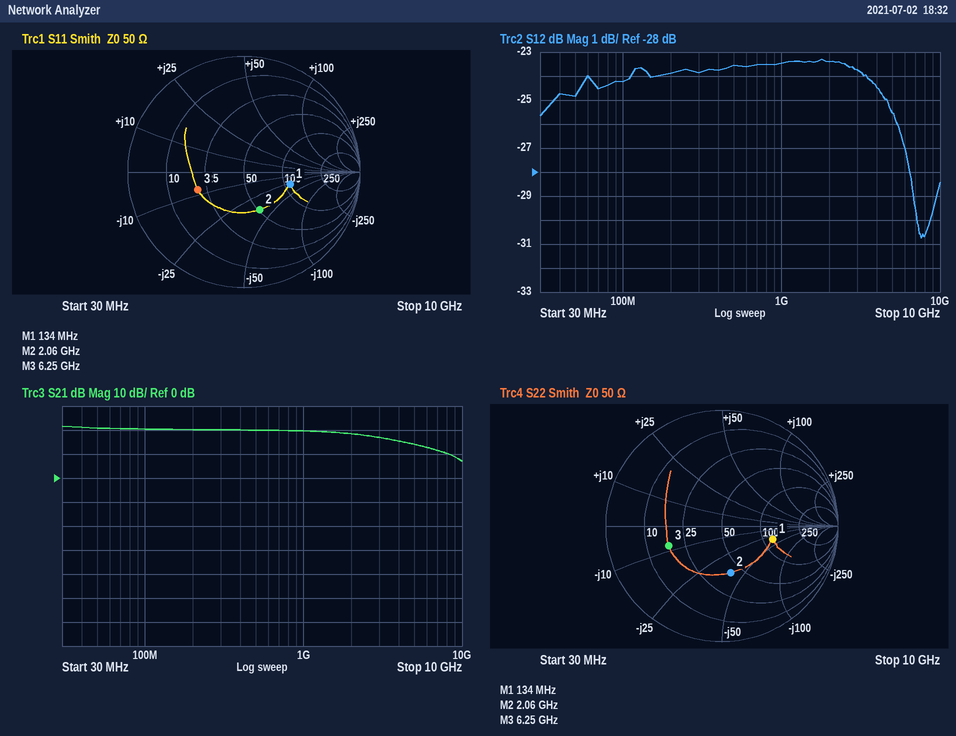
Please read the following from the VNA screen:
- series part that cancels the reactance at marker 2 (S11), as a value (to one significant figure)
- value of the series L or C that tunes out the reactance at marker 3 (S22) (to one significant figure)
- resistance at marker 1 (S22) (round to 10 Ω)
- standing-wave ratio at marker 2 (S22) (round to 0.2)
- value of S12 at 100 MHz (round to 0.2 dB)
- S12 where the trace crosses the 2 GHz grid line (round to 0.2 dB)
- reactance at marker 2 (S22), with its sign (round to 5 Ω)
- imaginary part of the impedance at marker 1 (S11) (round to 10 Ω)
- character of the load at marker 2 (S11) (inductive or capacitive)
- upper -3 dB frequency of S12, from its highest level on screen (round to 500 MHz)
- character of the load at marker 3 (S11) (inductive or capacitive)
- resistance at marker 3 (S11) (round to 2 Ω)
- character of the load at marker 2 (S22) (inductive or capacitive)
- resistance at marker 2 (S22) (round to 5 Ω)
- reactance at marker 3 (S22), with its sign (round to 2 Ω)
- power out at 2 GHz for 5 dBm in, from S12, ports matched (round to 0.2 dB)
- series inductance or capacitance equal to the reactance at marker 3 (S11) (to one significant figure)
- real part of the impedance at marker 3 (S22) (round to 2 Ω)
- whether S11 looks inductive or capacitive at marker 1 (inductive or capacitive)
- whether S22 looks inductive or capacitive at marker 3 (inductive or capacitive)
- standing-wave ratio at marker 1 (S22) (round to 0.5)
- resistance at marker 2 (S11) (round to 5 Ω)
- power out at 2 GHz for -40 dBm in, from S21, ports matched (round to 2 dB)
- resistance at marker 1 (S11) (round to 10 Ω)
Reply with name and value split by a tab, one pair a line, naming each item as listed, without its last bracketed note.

series part that cancels the reactance at marker 2 (S11), as a value	3 nH
value of the series L or C that tunes out the reactance at marker 3 (S22)	200 pH
resistance at marker 1 (S22)	120 Ω
standing-wave ratio at marker 2 (S22)	2.4
value of S12 at 100 MHz	-24.2 dB
S12 where the trace crosses the 2 GHz grid line	-23.4 dB
reactance at marker 2 (S22), with its sign	-40 Ω
imaginary part of the impedance at marker 1 (S11)	-30 Ω
character of the load at marker 2 (S11)	capacitive
upper -3 dB frequency of S12, from its highest level on screen	5.5 GHz
character of the load at marker 3 (S11)	capacitive
resistance at marker 3 (S11)	20 Ω
character of the load at marker 2 (S22)	capacitive
resistance at marker 2 (S22)	40 Ω
reactance at marker 3 (S22), with its sign	-8 Ω
power out at 2 GHz for 5 dBm in, from S12, ports matched	-18.4 dBm
series inductance or capacitance equal to the reactance at marker 3 (S11)	3 pF
real part of the impedance at marker 3 (S22)	18 Ω
whether S11 looks inductive or capacitive at marker 1	capacitive
whether S22 looks inductive or capacitive at marker 3	capacitive
standing-wave ratio at marker 1 (S22)	2.5
resistance at marker 2 (S11)	50 Ω
power out at 2 GHz for -40 dBm in, from S21, ports matched	-22 dBm
resistance at marker 1 (S11)	110 Ω
